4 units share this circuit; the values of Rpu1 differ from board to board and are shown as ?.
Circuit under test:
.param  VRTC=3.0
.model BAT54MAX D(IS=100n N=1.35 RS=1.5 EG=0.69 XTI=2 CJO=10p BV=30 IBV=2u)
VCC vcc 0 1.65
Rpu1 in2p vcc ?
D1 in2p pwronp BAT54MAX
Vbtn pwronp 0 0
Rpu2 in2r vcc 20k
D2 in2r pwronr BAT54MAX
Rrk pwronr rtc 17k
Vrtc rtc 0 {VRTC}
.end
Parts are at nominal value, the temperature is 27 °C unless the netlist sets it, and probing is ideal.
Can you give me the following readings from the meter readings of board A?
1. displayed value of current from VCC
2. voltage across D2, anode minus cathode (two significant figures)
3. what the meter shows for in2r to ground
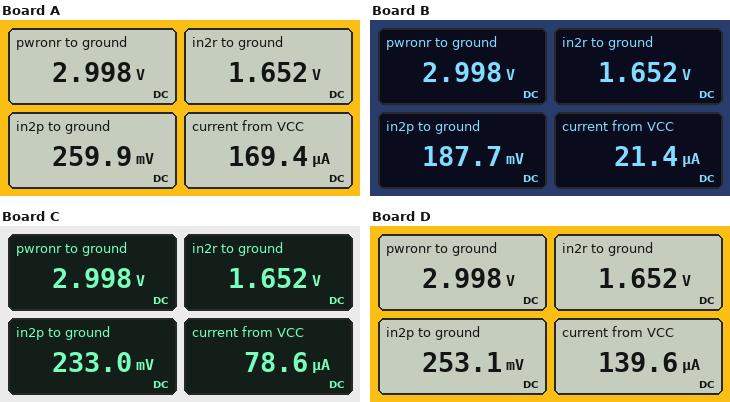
169.4 µA
-1.3 V
1.652 V
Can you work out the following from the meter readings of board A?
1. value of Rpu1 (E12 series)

8.2 kΩ
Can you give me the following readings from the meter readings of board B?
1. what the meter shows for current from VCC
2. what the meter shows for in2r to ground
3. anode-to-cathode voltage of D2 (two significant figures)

21.4 µA
1.652 V
-1.3 V
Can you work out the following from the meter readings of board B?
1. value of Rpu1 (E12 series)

68 kΩ
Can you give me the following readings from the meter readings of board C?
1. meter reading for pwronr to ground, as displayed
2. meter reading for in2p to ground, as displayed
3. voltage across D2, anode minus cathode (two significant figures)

2.998 V
233.0 mV
-1.3 V
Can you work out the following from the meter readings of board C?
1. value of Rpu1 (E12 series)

18 kΩ
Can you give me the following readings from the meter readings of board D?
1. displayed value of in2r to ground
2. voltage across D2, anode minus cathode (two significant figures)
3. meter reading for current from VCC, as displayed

1.652 V
-1.3 V
139.6 µA
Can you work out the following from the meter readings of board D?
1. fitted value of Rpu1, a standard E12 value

10 kΩ
